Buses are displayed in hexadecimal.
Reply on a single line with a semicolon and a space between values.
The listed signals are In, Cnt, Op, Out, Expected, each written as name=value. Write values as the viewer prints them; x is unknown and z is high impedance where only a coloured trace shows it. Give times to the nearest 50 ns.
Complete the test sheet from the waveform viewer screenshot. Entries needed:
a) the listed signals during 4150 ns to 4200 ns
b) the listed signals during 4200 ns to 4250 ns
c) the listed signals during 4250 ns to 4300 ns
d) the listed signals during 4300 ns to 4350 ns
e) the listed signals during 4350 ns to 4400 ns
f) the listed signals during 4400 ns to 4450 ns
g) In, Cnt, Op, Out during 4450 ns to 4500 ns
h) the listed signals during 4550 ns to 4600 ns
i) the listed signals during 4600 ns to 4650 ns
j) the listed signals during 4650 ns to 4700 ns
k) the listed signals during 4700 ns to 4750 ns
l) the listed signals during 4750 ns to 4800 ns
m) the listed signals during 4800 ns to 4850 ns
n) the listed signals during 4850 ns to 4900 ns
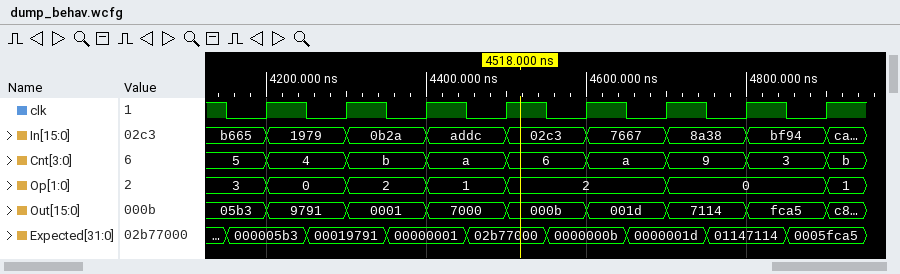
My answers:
In=b665, Cnt=5, Op=3, Out=05b3, Expected=000005b3; In=1979, Cnt=4, Op=0, Out=9791, Expected=000005b3; In=1979, Cnt=4, Op=0, Out=9791, Expected=00019791; In=0b2a, Cnt=b, Op=2, Out=0001, Expected=00019791; In=0b2a, Cnt=b, Op=2, Out=0001, Expected=00000001; In=addc, Cnt=a, Op=1, Out=7000, Expected=00000001; In=addc, Cnt=a, Op=1, Out=7000; In=02c3, Cnt=6, Op=2, Out=000b, Expected=0000000b; In=7667, Cnt=a, Op=2, Out=001d, Expected=0000000b; In=7667, Cnt=a, Op=2, Out=001d, Expected=0000001d; In=8a38, Cnt=9, Op=0, Out=7114, Expected=0000001d; In=8a38, Cnt=9, Op=0, Out=7114, Expected=01147114; In=bf94, Cnt=3, Op=0, Out=fca5, Expected=01147114; In=bf94, Cnt=3, Op=0, Out=fca5, Expected=0005fca5
